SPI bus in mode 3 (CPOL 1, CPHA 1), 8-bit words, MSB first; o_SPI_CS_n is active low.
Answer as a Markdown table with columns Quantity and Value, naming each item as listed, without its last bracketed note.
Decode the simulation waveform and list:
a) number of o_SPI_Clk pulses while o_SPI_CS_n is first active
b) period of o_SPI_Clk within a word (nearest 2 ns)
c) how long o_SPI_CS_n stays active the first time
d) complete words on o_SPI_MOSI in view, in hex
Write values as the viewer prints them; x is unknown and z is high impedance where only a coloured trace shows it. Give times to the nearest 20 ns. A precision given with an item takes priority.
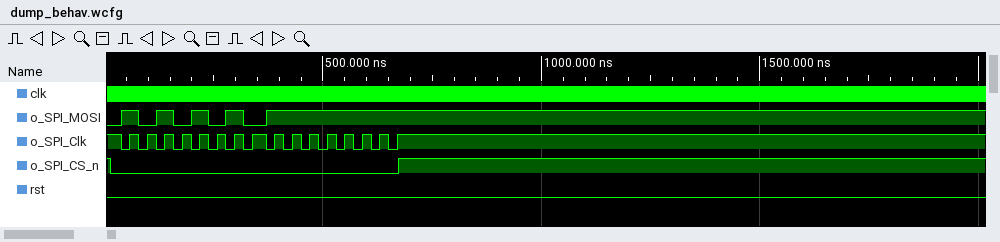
| Quantity | Value |
|---|---|
| number of o_SPI_Clk pulses while o_SPI_CS_n is first active | 16 |
| period of o_SPI_Clk within a word | 40 ns |
| how long o_SPI_CS_n stays active the first time | 660 ns |
| complete words on o_SPI_MOSI in view, in hex | AA, FF |
